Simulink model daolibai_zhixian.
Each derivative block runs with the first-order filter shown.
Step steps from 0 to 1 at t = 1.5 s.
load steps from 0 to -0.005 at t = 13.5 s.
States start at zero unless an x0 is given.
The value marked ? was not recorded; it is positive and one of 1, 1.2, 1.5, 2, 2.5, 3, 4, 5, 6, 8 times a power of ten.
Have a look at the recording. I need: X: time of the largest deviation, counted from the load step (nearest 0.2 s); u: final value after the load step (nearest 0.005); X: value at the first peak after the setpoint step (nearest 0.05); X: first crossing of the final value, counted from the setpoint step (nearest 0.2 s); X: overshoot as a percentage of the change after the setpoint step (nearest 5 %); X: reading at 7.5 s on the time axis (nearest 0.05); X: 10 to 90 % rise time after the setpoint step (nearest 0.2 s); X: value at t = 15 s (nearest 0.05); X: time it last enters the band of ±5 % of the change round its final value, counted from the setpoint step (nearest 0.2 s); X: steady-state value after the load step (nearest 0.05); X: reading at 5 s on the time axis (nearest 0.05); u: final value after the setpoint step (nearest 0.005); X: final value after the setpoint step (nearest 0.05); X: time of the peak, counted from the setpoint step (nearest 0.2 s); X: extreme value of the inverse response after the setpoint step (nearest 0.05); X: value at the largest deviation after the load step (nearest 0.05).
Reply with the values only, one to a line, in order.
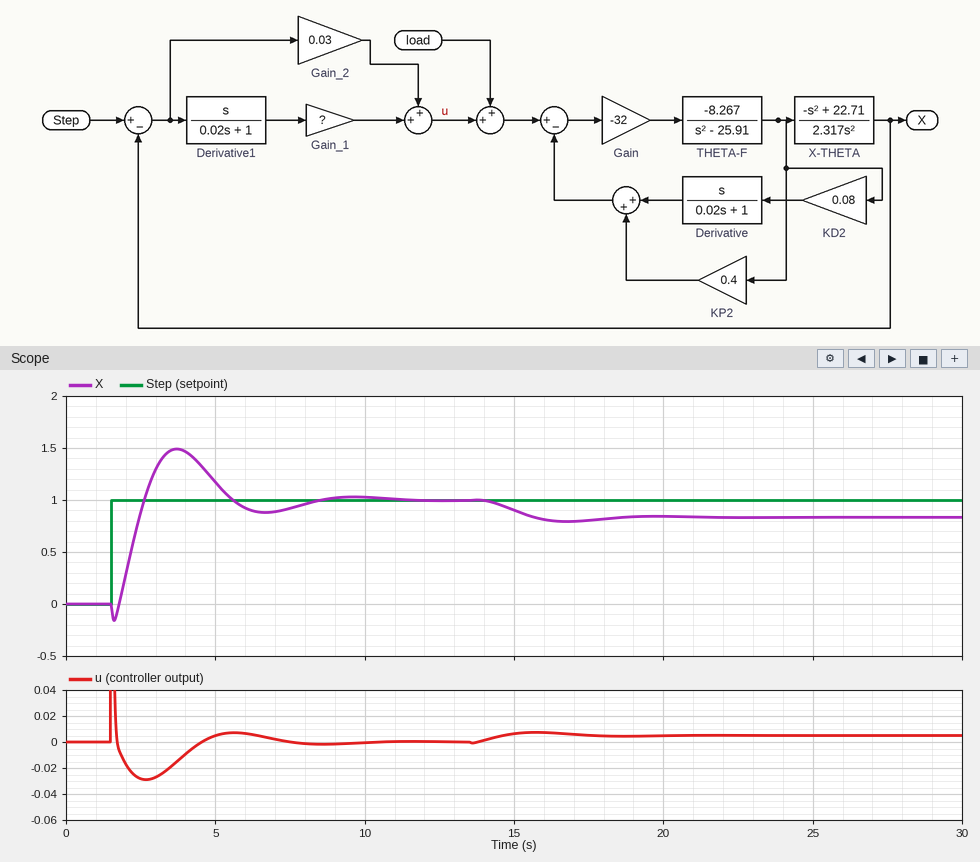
3.2 s
0.005
1.50
1.2 s
50 %
0.90
0.6 s
0.90
6.4 s
0.85
1.15
0.000
1.00
2.2 s
-0.15
0.80
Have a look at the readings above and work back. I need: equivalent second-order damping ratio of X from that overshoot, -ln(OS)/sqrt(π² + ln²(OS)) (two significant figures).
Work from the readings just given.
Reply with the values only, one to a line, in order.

0.22
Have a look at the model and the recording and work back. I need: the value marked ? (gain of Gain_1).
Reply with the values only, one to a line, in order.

0.03
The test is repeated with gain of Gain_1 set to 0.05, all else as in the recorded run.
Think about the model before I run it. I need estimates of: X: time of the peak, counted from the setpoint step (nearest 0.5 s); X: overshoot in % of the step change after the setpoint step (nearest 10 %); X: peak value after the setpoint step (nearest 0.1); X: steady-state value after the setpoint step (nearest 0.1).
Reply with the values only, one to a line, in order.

1.5 s
30 %
1.3
1.0
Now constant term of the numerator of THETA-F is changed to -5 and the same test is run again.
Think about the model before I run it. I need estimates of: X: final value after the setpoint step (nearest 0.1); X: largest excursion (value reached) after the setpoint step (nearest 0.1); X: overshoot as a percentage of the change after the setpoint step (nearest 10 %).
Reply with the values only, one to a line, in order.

1.0
1.6
60 %
